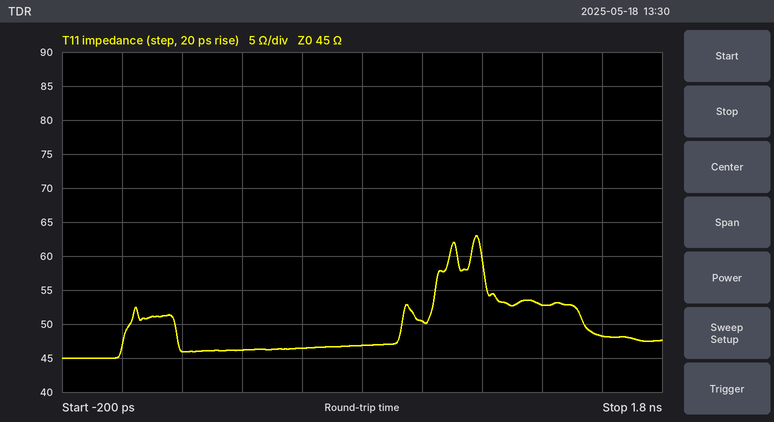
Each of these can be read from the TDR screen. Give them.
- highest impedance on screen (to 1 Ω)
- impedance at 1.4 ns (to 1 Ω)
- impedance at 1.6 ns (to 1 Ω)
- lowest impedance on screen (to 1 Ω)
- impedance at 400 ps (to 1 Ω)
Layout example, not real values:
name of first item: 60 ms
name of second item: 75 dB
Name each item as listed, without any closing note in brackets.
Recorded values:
highest impedance on screen: 63 Ω
impedance at 1.4 ns: 53 Ω
impedance at 1.6 ns: 48 Ω
lowest impedance on screen: 45 Ω
impedance at 400 ps: 46 Ω
